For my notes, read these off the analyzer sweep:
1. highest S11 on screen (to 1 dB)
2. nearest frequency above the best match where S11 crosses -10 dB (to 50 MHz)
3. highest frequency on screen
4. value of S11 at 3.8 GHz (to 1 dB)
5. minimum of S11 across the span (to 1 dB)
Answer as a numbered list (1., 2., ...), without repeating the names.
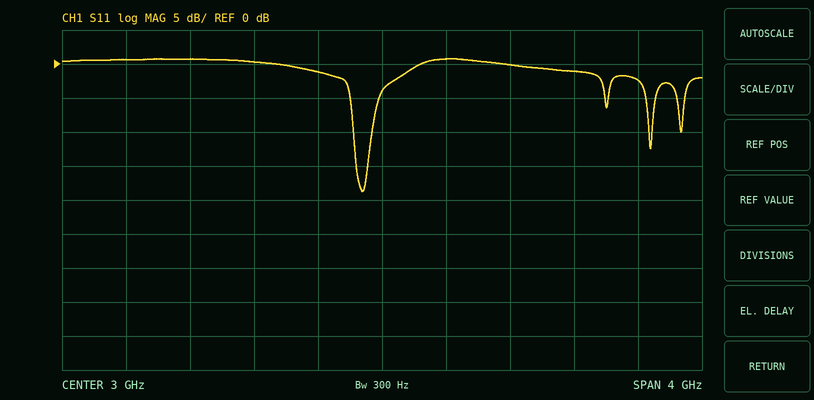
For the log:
1. 1 dB
2. 2.95 GHz
3. 5 GHz
4. 0 dB
5. -19 dB
